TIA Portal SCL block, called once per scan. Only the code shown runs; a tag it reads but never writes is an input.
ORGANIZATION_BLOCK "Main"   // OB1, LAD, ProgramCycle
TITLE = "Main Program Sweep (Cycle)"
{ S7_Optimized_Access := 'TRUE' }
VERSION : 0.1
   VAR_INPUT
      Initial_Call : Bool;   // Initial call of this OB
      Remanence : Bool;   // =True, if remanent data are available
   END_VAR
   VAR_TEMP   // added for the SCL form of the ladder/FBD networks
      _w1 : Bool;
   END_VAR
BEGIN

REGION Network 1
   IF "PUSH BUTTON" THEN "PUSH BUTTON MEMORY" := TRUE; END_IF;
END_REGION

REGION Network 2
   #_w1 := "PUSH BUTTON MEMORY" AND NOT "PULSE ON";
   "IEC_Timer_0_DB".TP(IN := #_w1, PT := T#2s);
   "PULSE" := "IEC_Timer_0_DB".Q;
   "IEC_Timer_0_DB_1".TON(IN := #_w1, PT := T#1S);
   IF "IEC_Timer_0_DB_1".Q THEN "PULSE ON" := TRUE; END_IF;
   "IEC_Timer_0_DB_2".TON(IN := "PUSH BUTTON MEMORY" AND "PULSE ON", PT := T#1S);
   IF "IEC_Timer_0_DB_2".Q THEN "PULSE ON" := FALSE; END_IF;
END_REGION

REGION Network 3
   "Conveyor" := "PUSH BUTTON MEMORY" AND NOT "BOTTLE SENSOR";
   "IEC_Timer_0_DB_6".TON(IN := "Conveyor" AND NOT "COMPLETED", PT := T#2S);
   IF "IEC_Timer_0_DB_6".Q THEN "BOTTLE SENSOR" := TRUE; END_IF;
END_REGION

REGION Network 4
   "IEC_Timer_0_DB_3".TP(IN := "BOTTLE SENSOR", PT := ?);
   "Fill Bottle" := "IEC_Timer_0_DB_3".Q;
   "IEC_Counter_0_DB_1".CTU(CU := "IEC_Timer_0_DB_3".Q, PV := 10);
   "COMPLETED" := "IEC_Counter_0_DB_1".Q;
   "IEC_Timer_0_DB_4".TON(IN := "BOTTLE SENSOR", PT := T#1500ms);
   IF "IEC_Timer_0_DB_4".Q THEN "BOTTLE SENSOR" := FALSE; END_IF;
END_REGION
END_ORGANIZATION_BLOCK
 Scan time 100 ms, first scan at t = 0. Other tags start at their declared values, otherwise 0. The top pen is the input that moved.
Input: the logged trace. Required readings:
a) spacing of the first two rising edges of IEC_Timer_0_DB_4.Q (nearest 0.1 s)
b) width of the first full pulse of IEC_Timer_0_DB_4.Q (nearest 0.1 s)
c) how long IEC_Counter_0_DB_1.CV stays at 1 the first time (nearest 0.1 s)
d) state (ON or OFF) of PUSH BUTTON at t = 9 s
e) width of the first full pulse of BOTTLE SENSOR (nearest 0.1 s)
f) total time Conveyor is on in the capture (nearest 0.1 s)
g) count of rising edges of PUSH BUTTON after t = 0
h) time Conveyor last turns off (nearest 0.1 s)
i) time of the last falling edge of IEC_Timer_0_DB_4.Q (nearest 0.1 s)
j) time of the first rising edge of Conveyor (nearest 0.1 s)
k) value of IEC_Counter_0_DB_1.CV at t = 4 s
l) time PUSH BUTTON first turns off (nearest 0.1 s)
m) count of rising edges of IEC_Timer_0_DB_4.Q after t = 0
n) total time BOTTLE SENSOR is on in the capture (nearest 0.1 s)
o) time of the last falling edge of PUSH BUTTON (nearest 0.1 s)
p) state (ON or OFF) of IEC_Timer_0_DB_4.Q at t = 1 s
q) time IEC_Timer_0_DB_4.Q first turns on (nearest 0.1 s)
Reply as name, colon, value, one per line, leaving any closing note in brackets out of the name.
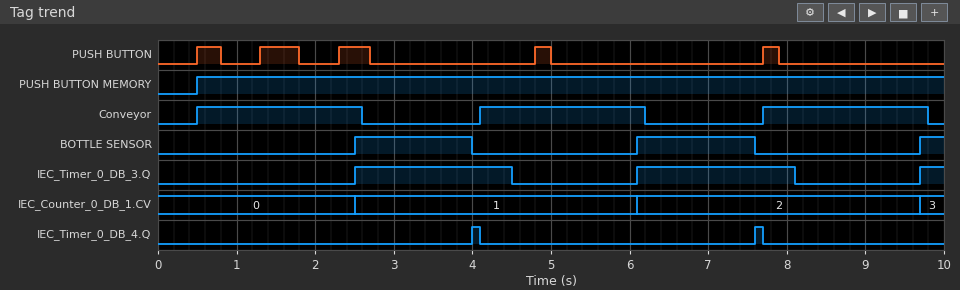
spacing of the first two rising edges of IEC_Timer_0_DB_4.Q: 3.6 s
width of the first full pulse of IEC_Timer_0_DB_4.Q: 0.1 s
how long IEC_Counter_0_DB_1.CV stays at 1 the first time: 3.6 s
state (ON or OFF) of PUSH BUTTON at t = 9 s: OFF
width of the first full pulse of BOTTLE SENSOR: 1.5 s
total time Conveyor is on in the capture: 6.3 s
count of rising edges of PUSH BUTTON after t = 0: 5
time Conveyor last turns off: 9.8 s
time of the last falling edge of IEC_Timer_0_DB_4.Q: 7.7 s
time of the first rising edge of Conveyor: 0.5 s
value of IEC_Counter_0_DB_1.CV at t = 4 s: 1
time PUSH BUTTON first turns off: 0.8 s
count of rising edges of IEC_Timer_0_DB_4.Q after t = 0: 2
total time BOTTLE SENSOR is on in the capture: 3.3 s
time of the last falling edge of PUSH BUTTON: 7.9 s
state (ON or OFF) of IEC_Timer_0_DB_4.Q at t = 1 s: OFF
time IEC_Timer_0_DB_4.Q first turns on: 4.0 s
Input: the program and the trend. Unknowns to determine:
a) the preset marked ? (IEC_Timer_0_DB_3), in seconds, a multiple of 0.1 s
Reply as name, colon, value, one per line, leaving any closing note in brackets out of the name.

the preset marked ? (IEC_Timer_0_DB_3), in seconds, a multiple of 0.1 s: 2.0 s
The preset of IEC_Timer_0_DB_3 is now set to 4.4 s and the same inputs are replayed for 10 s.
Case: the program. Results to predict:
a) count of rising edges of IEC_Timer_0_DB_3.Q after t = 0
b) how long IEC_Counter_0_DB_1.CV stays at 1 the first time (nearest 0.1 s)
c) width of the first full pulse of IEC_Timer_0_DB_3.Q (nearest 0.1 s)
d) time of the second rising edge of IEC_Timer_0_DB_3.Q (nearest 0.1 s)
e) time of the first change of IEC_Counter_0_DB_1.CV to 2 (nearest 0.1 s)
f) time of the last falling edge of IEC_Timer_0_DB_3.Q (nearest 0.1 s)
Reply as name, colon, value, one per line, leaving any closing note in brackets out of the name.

count of rising edges of IEC_Timer_0_DB_3.Q after t = 0: 2
how long IEC_Counter_0_DB_1.CV stays at 1 the first time: 7.2 s
width of the first full pulse of IEC_Timer_0_DB_3.Q: 4.4 s
time of the second rising edge of IEC_Timer_0_DB_3.Q: 9.7 s
time of the first change of IEC_Counter_0_DB_1.CV to 2: 9.7 s
time of the last falling edge of IEC_Timer_0_DB_3.Q: 6.9 s
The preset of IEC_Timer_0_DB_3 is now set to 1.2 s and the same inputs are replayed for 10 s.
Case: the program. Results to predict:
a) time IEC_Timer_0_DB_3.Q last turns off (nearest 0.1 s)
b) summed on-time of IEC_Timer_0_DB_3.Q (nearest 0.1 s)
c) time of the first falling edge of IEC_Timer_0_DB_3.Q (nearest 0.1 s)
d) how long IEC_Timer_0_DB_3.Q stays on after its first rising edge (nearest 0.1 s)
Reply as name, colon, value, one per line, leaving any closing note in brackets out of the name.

time IEC_Timer_0_DB_3.Q last turns off: 7.3 s
summed on-time of IEC_Timer_0_DB_3.Q: 2.7 s
time of the first falling edge of IEC_Timer_0_DB_3.Q: 3.7 s
how long IEC_Timer_0_DB_3.Q stays on after its first rising edge: 1.2 s
